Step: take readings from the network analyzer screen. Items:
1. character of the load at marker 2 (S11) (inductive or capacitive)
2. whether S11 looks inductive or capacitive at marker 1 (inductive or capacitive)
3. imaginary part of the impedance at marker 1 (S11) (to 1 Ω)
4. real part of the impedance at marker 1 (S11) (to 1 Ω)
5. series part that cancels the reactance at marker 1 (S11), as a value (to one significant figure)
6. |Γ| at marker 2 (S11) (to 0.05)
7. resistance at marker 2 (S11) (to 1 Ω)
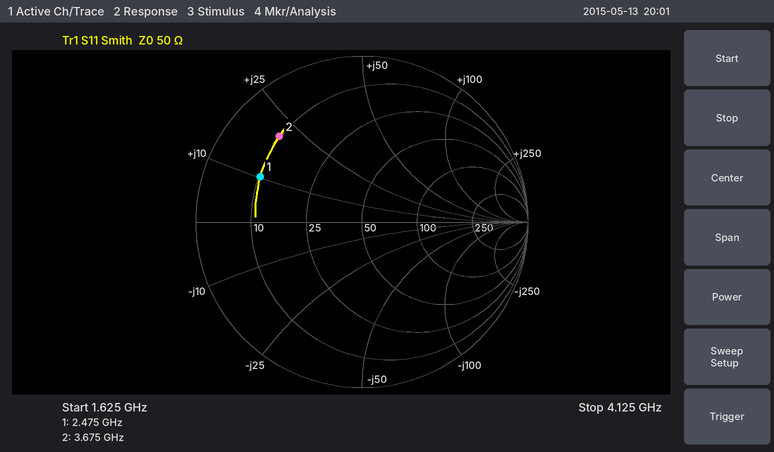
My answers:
inductive
inductive
+10 Ω
10 Ω
6 pF
0.70
10 Ω
